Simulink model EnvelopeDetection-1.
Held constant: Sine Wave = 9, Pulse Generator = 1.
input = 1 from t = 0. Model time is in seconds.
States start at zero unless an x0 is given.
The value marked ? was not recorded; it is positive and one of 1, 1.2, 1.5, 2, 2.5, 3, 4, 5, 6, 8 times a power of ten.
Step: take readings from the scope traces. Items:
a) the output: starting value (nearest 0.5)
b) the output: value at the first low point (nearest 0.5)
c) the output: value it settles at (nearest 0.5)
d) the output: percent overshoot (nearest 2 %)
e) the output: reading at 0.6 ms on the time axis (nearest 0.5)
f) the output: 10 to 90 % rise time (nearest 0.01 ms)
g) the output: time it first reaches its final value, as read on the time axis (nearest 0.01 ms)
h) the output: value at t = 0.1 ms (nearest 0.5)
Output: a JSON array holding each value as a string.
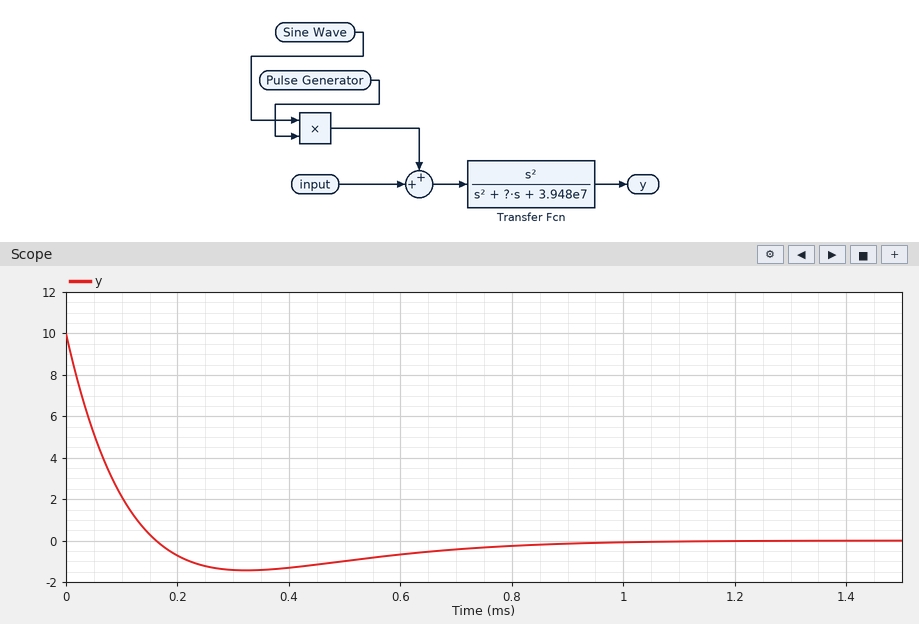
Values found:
["10.0", "-1.5", "0.0", "14 %", "-0.5", "0.12 ms", "0.16 ms", "2.0"]
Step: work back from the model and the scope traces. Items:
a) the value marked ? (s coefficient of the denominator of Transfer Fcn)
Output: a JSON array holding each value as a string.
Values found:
["12000"]
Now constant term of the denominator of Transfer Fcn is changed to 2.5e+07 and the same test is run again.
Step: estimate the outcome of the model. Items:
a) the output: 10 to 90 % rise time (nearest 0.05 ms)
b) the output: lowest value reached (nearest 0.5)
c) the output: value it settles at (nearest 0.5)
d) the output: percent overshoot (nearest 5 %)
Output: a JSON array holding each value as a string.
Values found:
["0.15 ms", "-1.0", "0.0", "10 %"]
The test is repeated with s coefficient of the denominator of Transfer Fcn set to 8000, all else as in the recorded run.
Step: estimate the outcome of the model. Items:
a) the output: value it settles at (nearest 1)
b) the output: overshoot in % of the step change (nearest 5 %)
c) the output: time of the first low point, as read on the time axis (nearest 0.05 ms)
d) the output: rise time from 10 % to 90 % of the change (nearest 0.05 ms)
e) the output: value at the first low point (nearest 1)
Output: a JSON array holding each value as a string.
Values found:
["0", "25 %", "0.35 ms", "0.15 ms", "-2"]
